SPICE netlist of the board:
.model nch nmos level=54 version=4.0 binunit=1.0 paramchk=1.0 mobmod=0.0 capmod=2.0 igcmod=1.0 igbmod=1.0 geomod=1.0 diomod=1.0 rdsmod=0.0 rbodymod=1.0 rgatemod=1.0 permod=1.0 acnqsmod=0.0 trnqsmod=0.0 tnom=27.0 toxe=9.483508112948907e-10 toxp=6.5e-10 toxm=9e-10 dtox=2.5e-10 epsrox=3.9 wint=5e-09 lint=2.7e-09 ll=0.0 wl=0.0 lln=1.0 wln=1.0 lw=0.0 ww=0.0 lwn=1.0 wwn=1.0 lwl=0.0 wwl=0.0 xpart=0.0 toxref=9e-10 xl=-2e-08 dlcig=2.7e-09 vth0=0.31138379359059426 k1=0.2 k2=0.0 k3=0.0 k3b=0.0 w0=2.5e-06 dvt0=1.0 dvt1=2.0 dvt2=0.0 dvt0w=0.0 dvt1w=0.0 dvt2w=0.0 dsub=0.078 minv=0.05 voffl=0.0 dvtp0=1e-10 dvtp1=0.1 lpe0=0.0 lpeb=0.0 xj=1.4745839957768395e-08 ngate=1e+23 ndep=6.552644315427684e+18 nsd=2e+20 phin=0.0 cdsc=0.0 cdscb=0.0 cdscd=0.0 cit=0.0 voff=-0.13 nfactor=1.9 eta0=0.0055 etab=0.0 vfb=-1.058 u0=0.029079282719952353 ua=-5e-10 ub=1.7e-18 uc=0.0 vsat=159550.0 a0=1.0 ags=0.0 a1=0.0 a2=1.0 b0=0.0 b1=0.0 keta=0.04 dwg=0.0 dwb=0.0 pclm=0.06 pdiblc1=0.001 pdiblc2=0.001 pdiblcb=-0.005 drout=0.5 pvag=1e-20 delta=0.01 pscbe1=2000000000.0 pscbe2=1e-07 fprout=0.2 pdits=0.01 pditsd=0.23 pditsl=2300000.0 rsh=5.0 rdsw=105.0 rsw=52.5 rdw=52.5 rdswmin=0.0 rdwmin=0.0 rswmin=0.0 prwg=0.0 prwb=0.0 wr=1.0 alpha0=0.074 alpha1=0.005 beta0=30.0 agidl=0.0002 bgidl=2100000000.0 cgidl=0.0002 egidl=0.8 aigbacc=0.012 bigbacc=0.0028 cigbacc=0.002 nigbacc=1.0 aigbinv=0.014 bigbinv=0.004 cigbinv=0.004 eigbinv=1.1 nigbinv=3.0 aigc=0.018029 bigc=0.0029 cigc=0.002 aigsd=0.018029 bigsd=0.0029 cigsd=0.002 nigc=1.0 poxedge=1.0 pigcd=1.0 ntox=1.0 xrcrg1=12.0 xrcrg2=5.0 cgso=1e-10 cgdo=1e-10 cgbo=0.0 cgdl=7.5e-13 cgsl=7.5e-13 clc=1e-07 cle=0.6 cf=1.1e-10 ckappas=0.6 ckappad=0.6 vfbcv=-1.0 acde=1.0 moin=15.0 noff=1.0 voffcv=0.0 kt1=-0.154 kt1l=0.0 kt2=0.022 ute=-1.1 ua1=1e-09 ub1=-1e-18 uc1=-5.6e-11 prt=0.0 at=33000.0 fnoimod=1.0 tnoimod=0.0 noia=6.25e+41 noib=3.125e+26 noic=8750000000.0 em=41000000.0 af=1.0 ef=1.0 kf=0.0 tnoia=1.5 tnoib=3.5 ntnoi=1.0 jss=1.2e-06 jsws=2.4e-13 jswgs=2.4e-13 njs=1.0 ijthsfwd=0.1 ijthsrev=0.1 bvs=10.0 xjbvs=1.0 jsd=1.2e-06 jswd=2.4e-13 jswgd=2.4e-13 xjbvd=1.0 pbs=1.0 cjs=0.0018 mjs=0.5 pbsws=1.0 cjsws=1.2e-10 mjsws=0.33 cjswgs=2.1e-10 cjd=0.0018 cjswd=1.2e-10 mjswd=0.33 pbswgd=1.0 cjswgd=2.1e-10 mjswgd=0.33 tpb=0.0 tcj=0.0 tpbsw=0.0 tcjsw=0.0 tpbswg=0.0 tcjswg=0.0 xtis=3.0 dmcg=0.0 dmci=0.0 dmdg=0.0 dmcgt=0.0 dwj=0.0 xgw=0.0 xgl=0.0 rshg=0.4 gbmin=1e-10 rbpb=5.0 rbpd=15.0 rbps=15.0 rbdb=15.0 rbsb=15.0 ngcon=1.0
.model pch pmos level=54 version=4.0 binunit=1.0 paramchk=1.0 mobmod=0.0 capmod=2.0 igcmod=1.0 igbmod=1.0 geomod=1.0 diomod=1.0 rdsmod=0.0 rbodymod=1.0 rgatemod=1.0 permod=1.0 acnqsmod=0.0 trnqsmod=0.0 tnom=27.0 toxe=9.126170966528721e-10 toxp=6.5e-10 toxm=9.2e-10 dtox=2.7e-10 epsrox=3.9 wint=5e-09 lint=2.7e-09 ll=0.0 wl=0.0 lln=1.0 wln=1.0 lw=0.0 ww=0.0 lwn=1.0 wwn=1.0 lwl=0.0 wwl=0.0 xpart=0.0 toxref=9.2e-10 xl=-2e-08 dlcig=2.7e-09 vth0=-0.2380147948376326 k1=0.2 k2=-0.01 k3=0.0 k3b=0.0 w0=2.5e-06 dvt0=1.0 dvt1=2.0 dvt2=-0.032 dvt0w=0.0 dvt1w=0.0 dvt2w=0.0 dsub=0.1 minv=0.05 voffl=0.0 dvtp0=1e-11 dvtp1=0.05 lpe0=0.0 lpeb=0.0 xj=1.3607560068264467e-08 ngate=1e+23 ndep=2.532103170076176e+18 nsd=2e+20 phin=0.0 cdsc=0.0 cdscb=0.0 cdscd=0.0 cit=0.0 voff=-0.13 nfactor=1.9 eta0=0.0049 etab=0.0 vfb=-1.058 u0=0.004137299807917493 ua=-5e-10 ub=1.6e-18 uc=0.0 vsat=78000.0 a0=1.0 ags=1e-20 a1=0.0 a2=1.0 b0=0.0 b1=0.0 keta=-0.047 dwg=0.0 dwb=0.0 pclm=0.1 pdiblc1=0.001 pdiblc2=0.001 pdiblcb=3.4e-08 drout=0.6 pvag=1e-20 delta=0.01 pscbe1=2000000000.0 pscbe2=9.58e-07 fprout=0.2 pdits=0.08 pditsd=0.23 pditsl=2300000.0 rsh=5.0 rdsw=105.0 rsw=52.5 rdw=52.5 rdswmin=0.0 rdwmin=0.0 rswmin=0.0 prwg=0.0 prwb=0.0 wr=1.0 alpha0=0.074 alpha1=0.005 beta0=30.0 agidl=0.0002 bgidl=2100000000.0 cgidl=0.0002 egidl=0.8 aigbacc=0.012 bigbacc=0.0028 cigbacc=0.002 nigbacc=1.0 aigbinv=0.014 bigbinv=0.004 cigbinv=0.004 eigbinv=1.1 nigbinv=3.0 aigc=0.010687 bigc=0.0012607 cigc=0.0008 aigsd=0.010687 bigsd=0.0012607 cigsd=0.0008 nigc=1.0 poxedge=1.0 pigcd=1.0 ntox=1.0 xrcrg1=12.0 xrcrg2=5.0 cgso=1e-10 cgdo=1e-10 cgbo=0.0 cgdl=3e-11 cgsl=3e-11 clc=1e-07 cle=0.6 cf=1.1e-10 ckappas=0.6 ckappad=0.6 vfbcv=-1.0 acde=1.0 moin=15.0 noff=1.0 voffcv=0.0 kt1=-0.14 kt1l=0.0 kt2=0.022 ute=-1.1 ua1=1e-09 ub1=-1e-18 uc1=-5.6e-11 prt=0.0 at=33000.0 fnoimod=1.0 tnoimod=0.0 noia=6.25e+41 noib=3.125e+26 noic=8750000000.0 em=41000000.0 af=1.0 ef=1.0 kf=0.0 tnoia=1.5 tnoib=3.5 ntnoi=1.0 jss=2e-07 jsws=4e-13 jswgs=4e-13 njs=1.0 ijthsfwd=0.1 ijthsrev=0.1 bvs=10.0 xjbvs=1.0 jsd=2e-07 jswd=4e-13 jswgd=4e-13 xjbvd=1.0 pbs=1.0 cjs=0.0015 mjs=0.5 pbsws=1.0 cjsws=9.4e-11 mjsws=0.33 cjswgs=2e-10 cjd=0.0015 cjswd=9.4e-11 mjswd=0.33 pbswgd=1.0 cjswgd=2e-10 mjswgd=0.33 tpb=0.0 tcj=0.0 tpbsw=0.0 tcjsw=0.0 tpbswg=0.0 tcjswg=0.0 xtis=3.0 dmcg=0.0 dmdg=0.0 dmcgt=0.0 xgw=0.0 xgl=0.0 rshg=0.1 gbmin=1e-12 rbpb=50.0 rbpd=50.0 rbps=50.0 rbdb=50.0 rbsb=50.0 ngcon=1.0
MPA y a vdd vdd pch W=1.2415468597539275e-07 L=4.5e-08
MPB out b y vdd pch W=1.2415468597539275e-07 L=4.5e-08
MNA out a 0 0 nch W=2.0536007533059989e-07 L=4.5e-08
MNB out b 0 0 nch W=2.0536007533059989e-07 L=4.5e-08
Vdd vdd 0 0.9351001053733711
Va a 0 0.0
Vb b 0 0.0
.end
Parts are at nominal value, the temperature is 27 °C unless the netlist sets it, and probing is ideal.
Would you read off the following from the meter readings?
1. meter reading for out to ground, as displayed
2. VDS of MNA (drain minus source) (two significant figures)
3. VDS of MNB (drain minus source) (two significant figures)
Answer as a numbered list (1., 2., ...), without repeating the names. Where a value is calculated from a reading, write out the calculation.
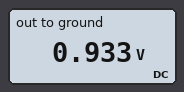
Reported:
1. 0.933 V
2. 933 mV = 930 mV
3. 933 mV = 930 mV
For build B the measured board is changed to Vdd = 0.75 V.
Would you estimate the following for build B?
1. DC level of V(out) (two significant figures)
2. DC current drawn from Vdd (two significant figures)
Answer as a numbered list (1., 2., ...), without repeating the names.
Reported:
1. 750 mV
2. 120 nA
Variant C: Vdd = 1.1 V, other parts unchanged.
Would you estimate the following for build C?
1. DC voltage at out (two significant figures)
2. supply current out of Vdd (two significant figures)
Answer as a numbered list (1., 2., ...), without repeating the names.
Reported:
1. 1.1 V
2. 350 nA
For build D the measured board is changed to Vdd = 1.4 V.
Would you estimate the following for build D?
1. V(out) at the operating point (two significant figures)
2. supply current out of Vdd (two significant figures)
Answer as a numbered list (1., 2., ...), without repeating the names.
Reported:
1. 1.4 V
2. 1.7 µA
